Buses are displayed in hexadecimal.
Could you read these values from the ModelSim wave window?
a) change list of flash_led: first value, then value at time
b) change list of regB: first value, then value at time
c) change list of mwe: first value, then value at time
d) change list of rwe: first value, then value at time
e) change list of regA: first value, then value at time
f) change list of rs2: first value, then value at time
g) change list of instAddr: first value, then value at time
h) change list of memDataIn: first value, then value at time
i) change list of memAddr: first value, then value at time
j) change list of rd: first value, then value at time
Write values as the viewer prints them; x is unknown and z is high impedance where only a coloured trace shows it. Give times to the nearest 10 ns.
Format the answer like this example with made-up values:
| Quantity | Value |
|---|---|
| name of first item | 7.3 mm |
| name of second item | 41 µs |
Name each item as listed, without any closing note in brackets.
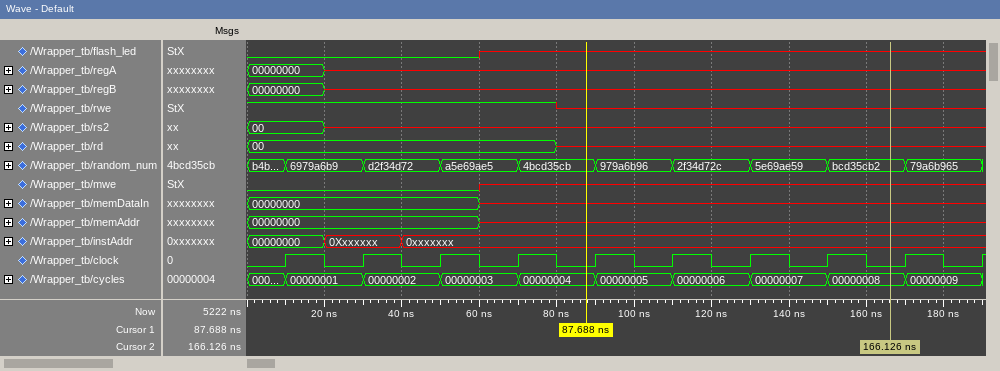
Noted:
| Quantity | Value |
|---|---|
| change list of flash_led: first value, then value at time | 0, x at 60 ns |
| change list of regB: first value, then value at time | 00000000, x at 20 ns |
| change list of mwe: first value, then value at time | 0, x at 60 ns |
| change list of rwe: first value, then value at time | 1, x at 80 ns |
| change list of regA: first value, then value at time | 00000000, x at 20 ns |
| change list of rs2: first value, then value at time | 00, x at 20 ns |
| change list of instAddr: first value, then value at time | 00000000, 0Xxxxxxx at 20 ns, 0xxxxxxx at 40 ns |
| change list of memDataIn: first value, then value at time | 00000000, x at 60 ns |
| change list of memAddr: first value, then value at time | 00000000, x at 60 ns |
| change list of rd: first value, then value at time | 00, x at 80 ns |
